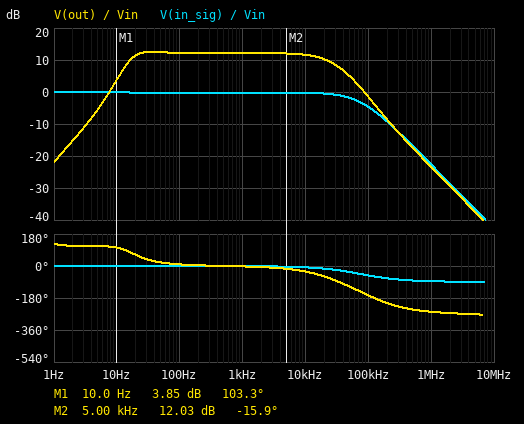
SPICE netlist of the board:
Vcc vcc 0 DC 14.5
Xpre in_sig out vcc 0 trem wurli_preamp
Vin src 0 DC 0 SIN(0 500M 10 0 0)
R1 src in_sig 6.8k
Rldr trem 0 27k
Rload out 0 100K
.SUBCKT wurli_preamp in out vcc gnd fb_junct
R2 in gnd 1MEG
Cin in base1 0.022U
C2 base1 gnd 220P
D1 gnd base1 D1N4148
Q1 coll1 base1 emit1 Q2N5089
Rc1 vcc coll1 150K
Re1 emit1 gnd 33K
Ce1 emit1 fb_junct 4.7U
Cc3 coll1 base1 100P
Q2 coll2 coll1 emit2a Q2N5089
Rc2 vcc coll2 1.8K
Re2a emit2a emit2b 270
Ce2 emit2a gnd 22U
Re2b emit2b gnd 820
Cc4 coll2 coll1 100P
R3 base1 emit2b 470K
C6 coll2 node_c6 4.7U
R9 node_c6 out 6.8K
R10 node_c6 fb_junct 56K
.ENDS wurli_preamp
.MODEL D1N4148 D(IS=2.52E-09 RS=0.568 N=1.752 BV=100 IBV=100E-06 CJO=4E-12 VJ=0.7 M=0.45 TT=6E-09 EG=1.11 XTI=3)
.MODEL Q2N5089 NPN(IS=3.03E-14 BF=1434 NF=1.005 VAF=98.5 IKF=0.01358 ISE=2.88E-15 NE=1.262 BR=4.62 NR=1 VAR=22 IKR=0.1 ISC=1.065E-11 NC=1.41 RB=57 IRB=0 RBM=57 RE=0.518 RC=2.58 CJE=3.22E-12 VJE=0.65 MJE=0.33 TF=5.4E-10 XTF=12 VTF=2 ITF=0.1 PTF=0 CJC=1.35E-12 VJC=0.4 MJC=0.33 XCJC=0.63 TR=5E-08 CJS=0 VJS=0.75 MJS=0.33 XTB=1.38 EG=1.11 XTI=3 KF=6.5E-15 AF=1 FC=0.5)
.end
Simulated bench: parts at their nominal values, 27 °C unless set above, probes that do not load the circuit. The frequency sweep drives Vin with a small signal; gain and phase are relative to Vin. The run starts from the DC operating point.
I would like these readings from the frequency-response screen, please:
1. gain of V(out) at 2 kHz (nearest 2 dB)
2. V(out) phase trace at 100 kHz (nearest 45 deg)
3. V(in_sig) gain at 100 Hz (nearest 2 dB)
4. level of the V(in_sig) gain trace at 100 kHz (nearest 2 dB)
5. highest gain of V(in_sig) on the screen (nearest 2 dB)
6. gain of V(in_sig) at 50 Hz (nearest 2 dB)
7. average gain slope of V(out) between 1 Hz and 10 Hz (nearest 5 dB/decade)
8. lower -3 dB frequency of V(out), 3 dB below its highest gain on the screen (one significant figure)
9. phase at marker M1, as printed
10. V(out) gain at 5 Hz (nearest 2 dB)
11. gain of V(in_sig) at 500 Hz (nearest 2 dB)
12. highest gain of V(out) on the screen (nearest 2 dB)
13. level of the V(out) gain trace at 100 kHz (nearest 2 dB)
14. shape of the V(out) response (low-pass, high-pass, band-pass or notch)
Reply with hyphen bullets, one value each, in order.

- 12 dB
- -180 deg
- 0 dB
- -4 dB
- 0 dB
- 0 dB
- 25 dB/decade
- 20 Hz
- 103.3 deg
- -6 dB
- 0 dB
- 12 dB
- -2 dB
- band-pass
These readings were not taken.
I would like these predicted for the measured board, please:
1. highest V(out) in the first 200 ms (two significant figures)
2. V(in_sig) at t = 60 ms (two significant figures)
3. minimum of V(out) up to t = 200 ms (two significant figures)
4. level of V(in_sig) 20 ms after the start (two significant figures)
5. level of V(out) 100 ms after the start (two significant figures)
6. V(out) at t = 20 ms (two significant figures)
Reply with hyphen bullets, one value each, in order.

- 780 mV
- -290 mV
- -790 mV
- 470 mV
- 760 mV
- 330 mV
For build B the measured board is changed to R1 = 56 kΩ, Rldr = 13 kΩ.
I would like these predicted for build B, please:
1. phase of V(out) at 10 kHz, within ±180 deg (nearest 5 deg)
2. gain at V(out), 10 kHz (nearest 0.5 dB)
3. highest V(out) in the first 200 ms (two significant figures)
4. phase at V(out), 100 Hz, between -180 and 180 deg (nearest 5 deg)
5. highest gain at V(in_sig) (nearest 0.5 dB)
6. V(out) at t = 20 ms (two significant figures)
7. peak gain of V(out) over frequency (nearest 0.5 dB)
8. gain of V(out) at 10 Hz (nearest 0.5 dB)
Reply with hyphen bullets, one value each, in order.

- -65 deg
- 11.0 dB
- 860 mV
- 10 deg
- -0.5 dB
- 310 mV
- 15.0 dB
- 4.5 dB
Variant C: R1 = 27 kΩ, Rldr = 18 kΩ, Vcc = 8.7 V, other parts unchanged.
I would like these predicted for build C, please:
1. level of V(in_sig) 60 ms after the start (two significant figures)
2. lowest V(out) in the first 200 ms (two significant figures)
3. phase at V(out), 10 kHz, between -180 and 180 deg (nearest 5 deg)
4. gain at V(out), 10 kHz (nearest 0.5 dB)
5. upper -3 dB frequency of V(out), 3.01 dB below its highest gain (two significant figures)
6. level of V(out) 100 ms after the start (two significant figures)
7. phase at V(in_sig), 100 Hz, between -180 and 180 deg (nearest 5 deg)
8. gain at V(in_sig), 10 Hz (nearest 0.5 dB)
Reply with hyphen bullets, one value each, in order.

- -270 mV
- -860 mV
- -50 deg
- 12.0 dB
- 13 kHz
- 790 mV
- 0 deg
- -0.5 dB
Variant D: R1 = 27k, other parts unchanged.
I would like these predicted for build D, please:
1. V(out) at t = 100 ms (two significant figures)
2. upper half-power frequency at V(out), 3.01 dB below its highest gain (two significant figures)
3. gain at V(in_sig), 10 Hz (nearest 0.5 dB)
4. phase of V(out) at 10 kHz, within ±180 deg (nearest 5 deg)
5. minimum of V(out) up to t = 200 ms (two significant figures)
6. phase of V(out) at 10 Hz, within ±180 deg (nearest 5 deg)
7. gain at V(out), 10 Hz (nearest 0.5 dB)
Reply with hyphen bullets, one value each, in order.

- 740 mV
- 14 kHz
- -0.5 dB
- -50 deg
- -760 mV
- 100 deg
- 3.5 dB
